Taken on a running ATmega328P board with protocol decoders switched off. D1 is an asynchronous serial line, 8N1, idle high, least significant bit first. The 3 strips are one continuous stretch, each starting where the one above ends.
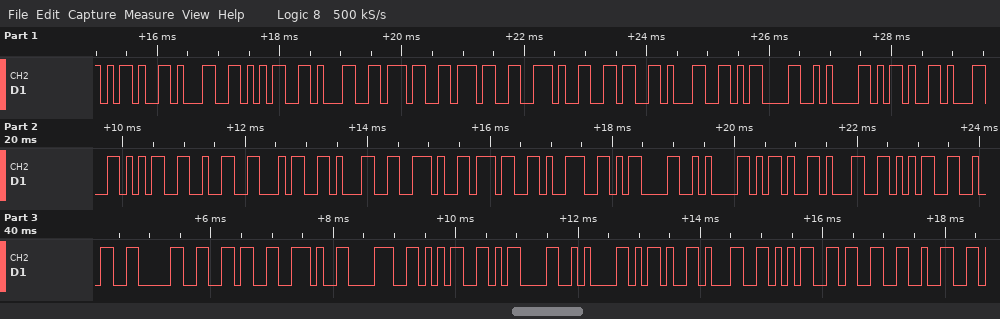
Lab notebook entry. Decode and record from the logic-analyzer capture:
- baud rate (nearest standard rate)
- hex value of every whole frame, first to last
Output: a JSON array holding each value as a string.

["9600 baud", "0x2D 0x31 0x35 0x31 0x37 0x37 0x2E 0x36 0x31 0x0D 0x0A 0x2D 0x31 0x35 0x32 0x34 0x31 0x2E 0x37 0x39 0x0D 0x0A 0x2D 0x31 0x35 0x32 0x30 0x36 0x2E 0x38 0x35 0x0D 0x0A 0x2D 0x31 0x35 0x33 0x32"]
